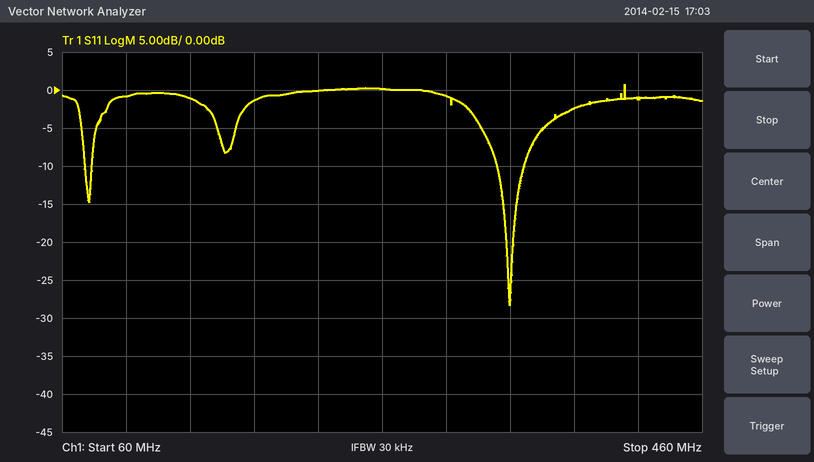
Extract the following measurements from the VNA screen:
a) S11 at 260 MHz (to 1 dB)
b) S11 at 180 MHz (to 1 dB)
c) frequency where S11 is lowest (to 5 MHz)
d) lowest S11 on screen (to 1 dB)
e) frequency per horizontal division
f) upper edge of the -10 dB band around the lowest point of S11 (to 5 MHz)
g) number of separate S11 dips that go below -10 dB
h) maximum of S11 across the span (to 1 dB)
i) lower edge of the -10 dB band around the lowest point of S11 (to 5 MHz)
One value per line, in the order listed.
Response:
0 dB
-1 dB
340 MHz
-28 dB
40 MHz
350 MHz
2
1 dB
330 MHz
